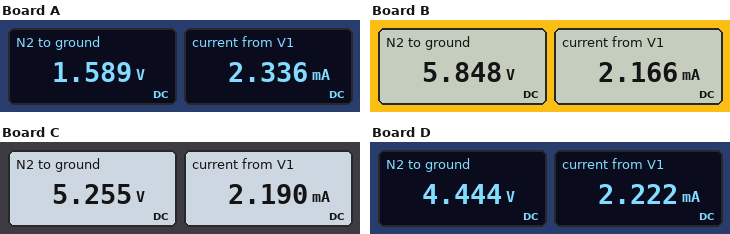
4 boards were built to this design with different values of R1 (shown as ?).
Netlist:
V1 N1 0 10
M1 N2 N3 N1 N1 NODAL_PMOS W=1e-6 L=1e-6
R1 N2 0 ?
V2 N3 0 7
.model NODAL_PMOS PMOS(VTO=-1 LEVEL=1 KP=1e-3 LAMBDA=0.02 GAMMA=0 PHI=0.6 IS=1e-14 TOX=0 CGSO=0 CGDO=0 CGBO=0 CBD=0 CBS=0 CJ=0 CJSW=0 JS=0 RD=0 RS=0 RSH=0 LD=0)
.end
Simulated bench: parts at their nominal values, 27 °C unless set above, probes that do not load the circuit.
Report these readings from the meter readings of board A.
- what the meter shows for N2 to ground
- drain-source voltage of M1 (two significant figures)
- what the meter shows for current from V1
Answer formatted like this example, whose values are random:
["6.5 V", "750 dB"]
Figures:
["1.589 V", "-8.4 V", "2.336 mA"]
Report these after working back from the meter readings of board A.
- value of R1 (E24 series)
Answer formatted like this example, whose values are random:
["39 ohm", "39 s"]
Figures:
["680 Ω"]
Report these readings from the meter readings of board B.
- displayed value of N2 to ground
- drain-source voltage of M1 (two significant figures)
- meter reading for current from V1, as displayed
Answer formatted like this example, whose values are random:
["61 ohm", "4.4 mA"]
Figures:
["5.848 V", "-4.2 V", "2.166 mA"]
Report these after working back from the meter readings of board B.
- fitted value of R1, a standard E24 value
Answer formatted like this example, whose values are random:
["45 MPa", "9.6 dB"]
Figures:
["2.7 kΩ"]
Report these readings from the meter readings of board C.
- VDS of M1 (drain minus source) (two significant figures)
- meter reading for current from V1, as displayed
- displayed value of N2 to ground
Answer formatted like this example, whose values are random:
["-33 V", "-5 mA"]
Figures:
["-4.7 V", "2.190 mA", "5.255 V"]
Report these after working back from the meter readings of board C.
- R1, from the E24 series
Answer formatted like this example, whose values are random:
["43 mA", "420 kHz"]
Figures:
["2.4 kΩ"]
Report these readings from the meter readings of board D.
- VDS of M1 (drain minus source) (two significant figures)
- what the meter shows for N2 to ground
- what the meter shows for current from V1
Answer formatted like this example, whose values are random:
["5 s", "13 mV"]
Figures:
["-5.6 V", "4.444 V", "2.222 mA"]
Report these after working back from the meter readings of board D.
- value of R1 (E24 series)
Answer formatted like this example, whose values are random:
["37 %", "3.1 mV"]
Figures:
["2 kΩ"]
